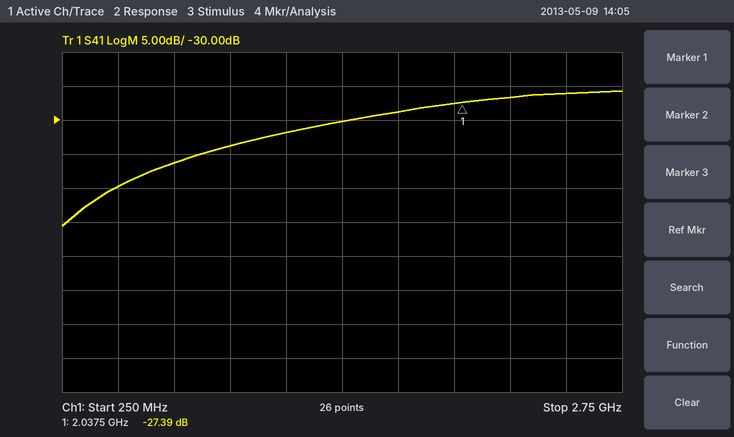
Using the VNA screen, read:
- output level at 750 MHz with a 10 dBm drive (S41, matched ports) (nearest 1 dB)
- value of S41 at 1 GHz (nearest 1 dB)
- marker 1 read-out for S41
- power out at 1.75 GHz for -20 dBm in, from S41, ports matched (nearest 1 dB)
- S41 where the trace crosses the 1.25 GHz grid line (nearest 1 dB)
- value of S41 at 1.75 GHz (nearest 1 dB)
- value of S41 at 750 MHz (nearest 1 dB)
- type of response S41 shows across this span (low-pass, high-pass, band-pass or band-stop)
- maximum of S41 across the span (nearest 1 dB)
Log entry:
-26 dBm
-34 dB
-27.39 dB
-49 dBm
-32 dB
-29 dB
-36 dB
high-pass
-26 dB
